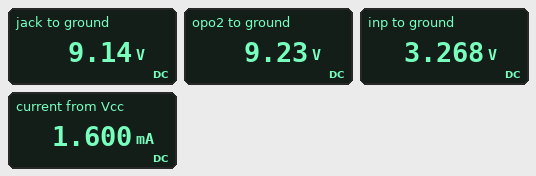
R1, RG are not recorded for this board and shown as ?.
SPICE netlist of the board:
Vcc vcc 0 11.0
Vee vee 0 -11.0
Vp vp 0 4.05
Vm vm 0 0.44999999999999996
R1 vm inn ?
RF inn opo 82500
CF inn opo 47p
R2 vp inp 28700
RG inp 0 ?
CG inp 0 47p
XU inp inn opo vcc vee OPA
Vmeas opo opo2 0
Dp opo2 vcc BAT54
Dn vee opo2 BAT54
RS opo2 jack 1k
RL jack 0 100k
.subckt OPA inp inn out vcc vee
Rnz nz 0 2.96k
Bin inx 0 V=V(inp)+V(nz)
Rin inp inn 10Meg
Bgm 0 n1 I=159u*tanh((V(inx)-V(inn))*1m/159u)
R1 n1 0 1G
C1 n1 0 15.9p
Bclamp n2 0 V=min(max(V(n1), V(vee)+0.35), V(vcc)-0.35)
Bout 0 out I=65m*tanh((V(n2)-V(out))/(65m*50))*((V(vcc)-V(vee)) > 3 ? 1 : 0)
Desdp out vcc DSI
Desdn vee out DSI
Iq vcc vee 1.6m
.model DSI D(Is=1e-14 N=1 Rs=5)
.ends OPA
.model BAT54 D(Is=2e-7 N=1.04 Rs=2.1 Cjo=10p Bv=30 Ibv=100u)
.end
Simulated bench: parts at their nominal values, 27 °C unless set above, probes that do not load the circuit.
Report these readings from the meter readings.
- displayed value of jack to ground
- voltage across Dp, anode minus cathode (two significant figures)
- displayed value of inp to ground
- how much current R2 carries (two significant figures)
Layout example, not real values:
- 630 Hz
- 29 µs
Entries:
- 9.14 V
- -1.8 V
- 3.268 V
- 27 µA
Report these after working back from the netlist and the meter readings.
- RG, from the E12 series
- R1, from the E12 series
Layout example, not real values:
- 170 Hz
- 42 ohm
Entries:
- 120 kΩ
- 39 kΩ
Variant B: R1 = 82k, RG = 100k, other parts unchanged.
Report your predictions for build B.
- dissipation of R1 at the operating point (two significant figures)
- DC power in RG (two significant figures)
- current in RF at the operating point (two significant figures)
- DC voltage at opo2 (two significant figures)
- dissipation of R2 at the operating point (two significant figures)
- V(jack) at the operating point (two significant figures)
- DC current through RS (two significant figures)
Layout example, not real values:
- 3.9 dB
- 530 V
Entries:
- 89 µW
- 99 µW
- 33 µA
- 5.9 V
- 28 µW
- 5.8 V
- 58 µA
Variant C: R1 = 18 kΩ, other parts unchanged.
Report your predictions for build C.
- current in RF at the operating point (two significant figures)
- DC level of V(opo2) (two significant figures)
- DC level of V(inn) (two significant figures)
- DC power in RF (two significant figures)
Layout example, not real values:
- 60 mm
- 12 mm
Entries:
- 100 µA
- 11 V
- 2.3 V
- 850 µW
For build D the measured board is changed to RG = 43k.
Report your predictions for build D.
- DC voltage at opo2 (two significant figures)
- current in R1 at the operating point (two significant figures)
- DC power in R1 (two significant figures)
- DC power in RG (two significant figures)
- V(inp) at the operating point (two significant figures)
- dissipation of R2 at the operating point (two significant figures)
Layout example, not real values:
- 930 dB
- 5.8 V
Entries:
- 6.6 V
- 51 µA
- 100 µW
- 140 µW
- 2.4 V
- 92 µW
